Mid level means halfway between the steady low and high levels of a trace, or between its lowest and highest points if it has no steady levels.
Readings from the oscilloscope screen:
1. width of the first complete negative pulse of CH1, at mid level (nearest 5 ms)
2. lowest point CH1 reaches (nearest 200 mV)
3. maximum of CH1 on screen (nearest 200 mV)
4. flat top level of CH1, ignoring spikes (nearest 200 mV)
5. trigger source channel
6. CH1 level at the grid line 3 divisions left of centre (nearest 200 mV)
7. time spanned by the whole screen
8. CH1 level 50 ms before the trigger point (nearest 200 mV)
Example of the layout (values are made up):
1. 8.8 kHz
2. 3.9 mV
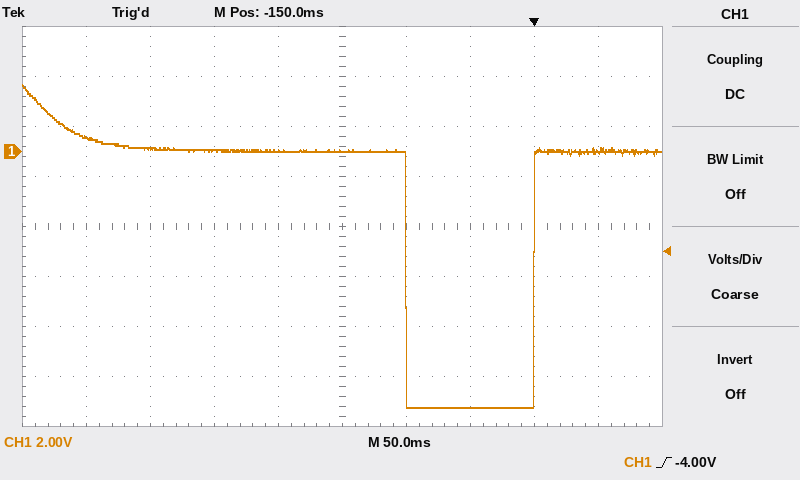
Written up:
1. 100 ms
2. -10.2 V
3. 2.6 V
4. 0.0 V
5. CH1
6. 200 mV
7. 500 ms
8. -10.2 V
